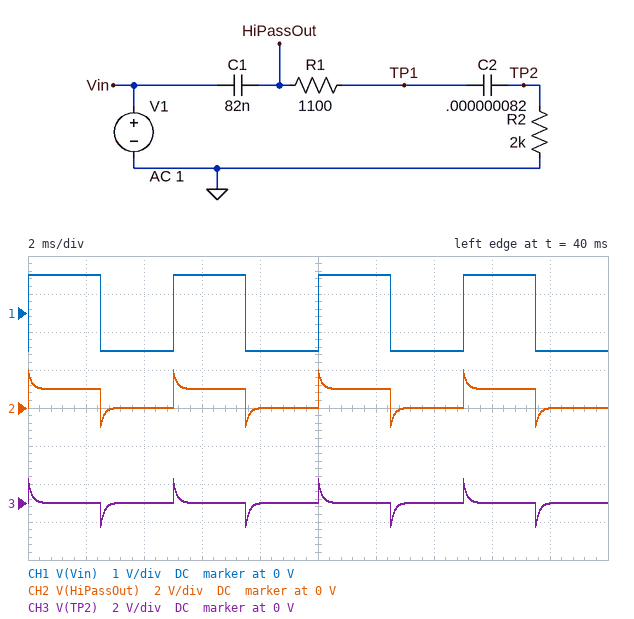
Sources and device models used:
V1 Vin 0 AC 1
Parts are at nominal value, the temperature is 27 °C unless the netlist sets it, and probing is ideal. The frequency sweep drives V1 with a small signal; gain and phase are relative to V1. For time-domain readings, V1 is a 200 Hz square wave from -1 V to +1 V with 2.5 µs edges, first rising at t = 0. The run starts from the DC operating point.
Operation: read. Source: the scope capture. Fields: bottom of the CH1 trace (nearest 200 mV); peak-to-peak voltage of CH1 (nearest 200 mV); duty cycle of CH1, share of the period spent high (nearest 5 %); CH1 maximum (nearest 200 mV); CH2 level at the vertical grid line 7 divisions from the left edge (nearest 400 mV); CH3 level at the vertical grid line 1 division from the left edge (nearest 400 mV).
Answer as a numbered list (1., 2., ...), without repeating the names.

1. -1.0 V
2. 2.0 V
3. 50 %
4. 1.0 V
5. 0 V
6. 0 V
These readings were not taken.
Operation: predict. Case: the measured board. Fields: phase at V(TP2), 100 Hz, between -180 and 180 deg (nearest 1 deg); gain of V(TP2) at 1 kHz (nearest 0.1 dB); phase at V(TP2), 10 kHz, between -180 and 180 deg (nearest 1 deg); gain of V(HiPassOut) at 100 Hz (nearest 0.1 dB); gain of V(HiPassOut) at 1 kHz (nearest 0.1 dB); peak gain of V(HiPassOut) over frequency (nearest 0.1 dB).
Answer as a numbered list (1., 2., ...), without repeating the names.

1. 85 deg
2. -7.9 dB
3. 7 deg
4. -5.9 dB
5. -2.7 dB
6. 0 dB
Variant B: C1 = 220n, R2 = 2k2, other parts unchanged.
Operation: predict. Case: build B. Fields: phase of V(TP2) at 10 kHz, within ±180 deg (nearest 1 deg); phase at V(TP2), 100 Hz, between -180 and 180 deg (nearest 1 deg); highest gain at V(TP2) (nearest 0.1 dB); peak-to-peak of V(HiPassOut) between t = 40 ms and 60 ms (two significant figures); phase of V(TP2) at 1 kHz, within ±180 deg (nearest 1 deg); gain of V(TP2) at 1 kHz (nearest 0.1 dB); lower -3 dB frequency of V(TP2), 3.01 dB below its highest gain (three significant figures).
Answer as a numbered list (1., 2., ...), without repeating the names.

1. 5 deg
2. 83 deg
3. -3.5 dB
4. 2.5 V
5. 39 deg
6. -5.7 dB
7. 807 Hz
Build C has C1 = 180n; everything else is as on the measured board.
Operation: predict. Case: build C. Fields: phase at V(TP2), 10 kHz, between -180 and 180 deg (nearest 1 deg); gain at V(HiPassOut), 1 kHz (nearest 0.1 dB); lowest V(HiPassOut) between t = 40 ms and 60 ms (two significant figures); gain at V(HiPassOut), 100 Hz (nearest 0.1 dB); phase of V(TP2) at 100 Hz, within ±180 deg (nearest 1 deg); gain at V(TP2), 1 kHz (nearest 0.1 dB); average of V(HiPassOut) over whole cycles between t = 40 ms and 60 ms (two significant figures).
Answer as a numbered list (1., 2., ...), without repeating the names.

1. 5 deg
2. -1.2 dB
3. -620 mV
4. -3.2 dB
5. 84 deg
6. -6.4 dB
7. 690 mV
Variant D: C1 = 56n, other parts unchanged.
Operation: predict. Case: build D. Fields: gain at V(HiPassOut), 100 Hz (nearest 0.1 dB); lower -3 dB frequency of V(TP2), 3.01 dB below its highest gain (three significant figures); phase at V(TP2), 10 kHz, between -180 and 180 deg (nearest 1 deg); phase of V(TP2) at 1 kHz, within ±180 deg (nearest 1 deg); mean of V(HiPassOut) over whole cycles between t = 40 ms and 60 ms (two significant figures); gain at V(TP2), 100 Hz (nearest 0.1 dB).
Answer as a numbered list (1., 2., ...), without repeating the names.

1. -7.7 dB
2. 1.54 kHz
3. 9 deg
4. 57 deg
5. 410 mV
6. -27.6 dB
